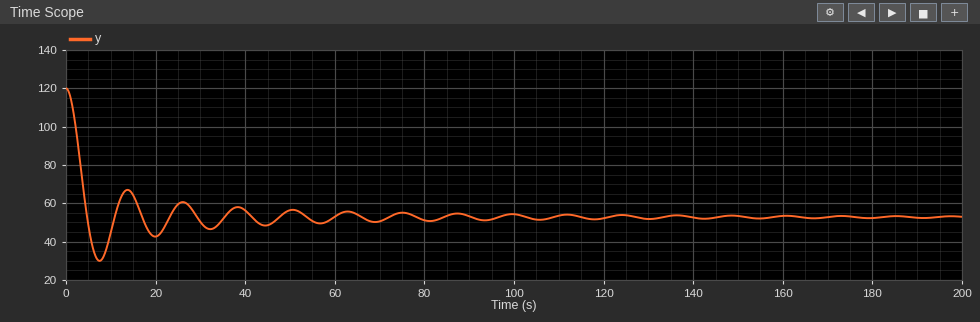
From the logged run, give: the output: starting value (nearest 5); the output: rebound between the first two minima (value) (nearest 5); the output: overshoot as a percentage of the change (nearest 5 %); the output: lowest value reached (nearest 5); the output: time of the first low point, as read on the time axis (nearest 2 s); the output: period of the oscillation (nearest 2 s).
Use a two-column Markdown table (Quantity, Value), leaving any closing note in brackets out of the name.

| Quantity | Value |
|---|---|
| the output: starting value | 120 |
| the output: rebound between the first two minima (value) | 65 |
| the output: overshoot as a percentage of the change | 35 % |
| the output: lowest value reached | 30 |
| the output: time of the first low point, as read on the time axis | 8 s |
| the output: period of the oscillation | 12 s |
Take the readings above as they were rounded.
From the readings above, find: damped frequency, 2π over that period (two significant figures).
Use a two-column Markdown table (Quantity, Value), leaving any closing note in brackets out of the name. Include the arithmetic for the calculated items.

| Quantity | Value |
|---|---|
| damped frequency, 2π over that period | 2π / 12 = 0.52 rad/s |
